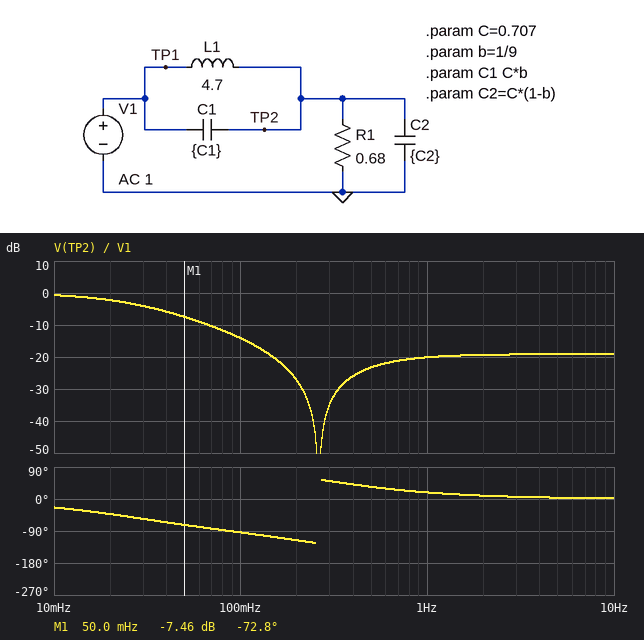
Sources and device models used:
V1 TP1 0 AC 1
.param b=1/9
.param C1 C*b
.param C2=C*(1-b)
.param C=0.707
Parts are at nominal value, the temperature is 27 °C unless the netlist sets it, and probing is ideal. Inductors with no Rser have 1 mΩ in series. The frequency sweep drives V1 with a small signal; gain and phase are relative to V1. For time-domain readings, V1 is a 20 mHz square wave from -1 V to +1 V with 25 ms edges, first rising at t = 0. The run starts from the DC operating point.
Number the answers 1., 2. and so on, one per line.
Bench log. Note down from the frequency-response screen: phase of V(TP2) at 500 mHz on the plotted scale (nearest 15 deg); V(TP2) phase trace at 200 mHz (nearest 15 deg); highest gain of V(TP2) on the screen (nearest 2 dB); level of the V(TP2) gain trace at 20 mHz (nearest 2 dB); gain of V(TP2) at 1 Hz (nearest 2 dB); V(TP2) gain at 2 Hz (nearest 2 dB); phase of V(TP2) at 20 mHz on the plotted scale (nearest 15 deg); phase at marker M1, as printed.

1. 30 deg
2. -120 deg
3. 0 dB
4. -2 dB
5. -20 dB
6. -20 dB
7. -45 deg
8. -72.8 deg
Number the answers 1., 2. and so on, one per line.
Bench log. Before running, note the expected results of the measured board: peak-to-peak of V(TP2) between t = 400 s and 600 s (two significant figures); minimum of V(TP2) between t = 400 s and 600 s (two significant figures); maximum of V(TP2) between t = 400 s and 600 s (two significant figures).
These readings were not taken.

1. 1.9 V
2. -960 mV
3. 960 mV
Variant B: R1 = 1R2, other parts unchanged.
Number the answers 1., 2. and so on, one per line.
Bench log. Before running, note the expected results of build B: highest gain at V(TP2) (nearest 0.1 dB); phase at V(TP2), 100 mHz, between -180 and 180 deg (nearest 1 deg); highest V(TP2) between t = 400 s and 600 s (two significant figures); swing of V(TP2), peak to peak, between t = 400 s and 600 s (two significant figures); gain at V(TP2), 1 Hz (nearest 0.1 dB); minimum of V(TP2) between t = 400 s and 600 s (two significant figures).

1. 0 dB
2. -97 deg
3. 1.0 V
4. 2.0 V
5. -19.8 dB
6. -1.0 V
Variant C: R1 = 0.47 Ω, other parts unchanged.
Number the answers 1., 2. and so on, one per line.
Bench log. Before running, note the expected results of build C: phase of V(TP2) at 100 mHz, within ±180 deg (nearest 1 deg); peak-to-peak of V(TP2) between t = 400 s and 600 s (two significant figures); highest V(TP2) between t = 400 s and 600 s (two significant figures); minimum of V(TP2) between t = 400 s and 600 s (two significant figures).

1. -93 deg
2. 1.7 V
3. 850 mV
4. -850 mV
